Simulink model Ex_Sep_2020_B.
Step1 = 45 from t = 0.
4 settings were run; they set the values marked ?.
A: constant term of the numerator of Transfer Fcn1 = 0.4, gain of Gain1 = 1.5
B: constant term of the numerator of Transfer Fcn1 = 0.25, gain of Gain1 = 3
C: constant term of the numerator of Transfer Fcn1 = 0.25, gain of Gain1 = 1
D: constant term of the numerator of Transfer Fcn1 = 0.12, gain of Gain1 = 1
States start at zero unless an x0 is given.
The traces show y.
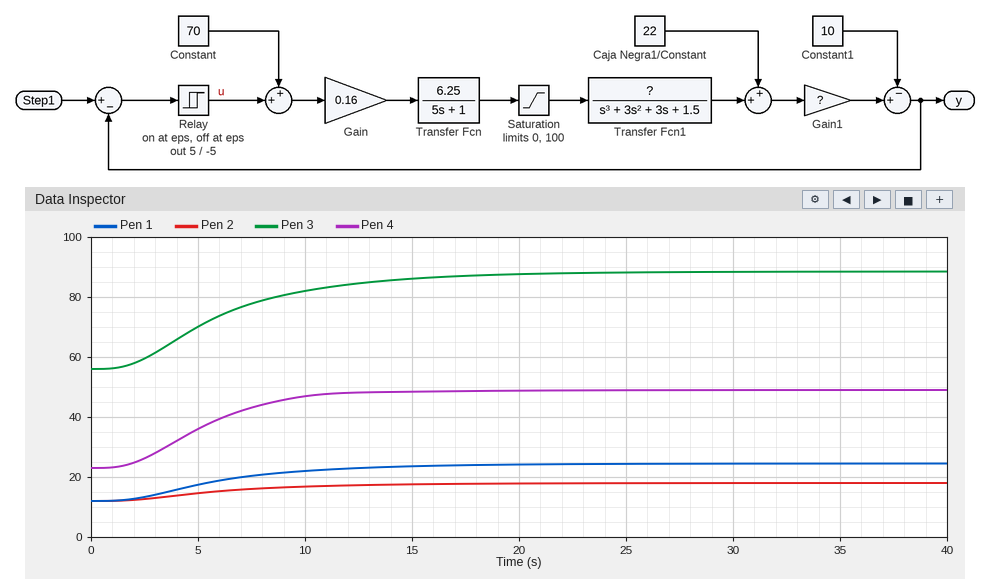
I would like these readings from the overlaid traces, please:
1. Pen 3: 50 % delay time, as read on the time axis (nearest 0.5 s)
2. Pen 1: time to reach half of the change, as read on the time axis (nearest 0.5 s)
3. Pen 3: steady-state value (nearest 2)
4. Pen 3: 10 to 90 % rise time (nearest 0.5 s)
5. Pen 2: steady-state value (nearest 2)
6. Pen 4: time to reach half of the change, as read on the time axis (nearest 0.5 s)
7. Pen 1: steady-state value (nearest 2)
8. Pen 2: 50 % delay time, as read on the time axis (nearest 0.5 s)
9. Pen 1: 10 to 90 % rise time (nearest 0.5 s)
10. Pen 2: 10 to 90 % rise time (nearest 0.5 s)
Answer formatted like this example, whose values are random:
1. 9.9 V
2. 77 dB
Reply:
1. 5.5 s
2. 5.5 s
3. 88
4. 11.0 s
5. 18
6. 5.0 s
7. 24
8. 5.5 s
9. 11.0 s
10. 11.0 s
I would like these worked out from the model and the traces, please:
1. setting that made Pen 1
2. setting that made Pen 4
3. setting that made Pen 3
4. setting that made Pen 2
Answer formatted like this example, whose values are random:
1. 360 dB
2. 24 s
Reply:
1. C
2. A
3. B
4. D
